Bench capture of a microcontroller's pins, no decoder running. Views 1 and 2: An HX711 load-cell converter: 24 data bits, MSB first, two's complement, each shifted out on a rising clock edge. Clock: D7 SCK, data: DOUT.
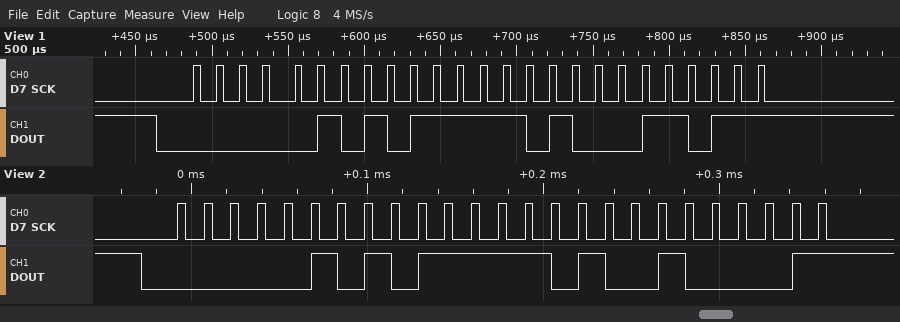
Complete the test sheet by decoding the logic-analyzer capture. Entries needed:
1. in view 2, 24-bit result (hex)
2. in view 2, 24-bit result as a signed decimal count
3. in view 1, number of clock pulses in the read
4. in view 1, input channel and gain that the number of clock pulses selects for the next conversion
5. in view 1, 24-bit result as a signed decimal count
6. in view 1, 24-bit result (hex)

0x057D21
359713
25
channel A, gain 128
359707
0x057D1B
